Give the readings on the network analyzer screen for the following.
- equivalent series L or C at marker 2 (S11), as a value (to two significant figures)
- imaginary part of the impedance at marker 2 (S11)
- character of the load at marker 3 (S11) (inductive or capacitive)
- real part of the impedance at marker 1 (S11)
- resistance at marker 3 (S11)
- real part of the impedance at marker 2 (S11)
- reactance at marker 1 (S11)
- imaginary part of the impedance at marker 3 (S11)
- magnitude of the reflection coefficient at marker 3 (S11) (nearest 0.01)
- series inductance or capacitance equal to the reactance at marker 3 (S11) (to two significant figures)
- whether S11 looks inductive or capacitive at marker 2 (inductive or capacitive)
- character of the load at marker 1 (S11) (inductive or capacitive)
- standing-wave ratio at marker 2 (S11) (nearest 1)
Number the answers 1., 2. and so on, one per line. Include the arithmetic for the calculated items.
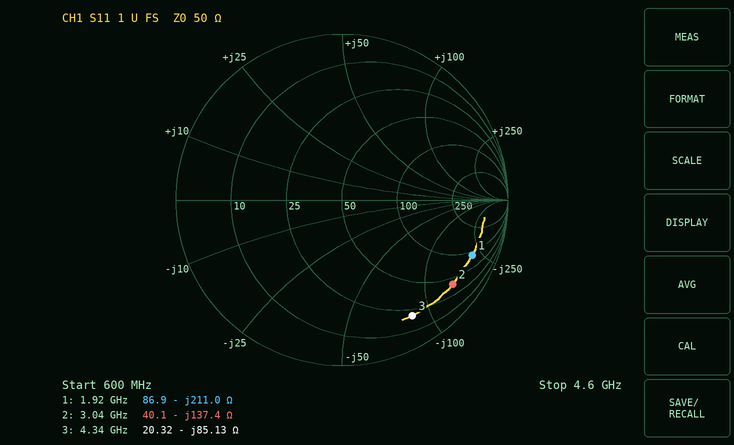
1. C = 1/(2π × 3.04 GHz × 137.4 Ω) ≈ 381 fF, so 380 fF to two significant figures
2. -137.4 Ω
3. capacitive
4. 86.9 Ω
5. 20.32 Ω
6. 40.1 Ω
7. -211.0 Ω
8. -85.13 Ω
9. 0.82
10. C = 1/(2π × 4.34 GHz × 85.13 Ω) ≈ 431 fF, so 430 fF to two significant figures
11. capacitive
12. capacitive
13. 11
